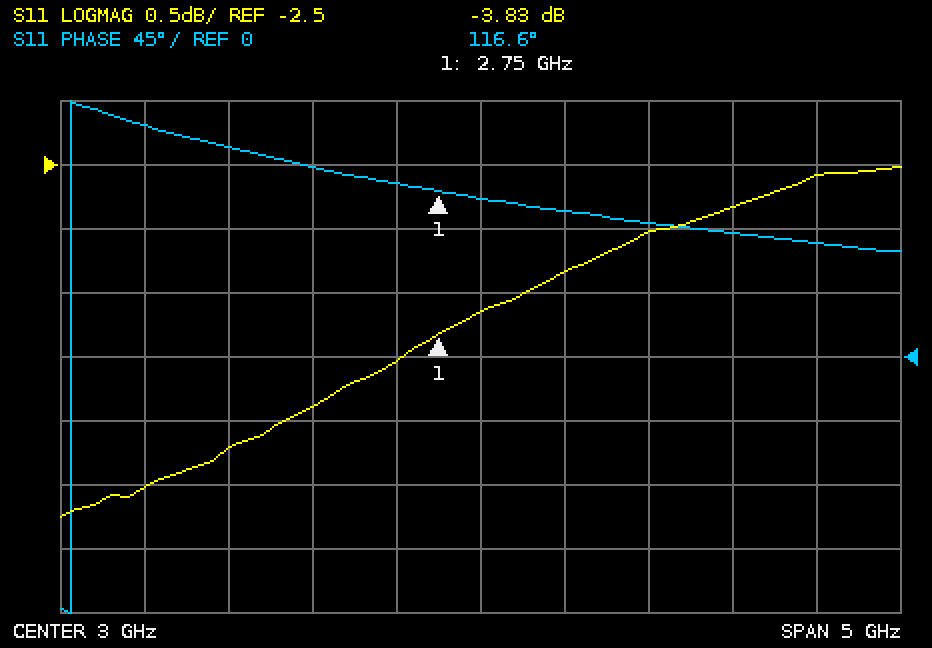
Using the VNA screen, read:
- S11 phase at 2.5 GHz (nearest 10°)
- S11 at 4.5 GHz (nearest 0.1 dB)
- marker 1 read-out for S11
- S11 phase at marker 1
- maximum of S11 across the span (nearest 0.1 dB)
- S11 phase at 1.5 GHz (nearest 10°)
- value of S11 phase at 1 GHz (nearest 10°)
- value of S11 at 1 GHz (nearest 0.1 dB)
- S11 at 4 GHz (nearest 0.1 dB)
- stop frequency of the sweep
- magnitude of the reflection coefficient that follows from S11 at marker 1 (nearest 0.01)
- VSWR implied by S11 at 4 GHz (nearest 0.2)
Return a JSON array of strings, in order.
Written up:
["120°", "-2.8 dB", "-3.83 dB", "116.6°", "-2.5 dB", "150°", "160°", "-5.0 dB", "-3.0 dB", "5.5 GHz", "0.64", "5.8"]
